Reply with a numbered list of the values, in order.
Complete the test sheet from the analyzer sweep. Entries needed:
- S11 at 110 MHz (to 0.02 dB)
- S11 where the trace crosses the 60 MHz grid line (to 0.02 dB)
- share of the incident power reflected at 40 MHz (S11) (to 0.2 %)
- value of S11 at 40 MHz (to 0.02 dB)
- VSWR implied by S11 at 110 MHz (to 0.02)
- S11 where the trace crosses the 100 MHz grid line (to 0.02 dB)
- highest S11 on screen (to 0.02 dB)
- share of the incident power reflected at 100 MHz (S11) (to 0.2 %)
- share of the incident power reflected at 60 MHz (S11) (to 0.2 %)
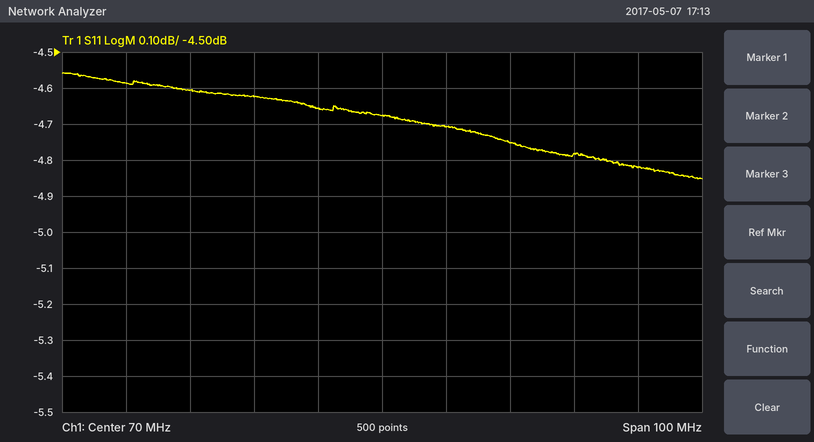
1. -4.82 dB
2. -4.66 dB
3. 34.6 %
4. -4.60 dB
5. 3.70
6. -4.78 dB
7. -4.56 dB
8. 33.2 %
9. 34.2 %
